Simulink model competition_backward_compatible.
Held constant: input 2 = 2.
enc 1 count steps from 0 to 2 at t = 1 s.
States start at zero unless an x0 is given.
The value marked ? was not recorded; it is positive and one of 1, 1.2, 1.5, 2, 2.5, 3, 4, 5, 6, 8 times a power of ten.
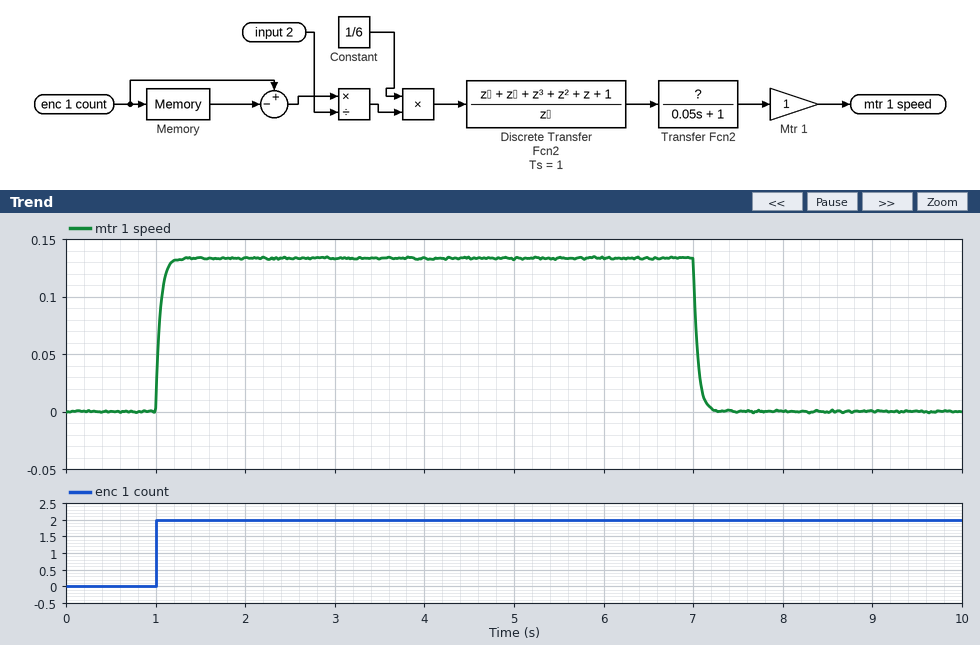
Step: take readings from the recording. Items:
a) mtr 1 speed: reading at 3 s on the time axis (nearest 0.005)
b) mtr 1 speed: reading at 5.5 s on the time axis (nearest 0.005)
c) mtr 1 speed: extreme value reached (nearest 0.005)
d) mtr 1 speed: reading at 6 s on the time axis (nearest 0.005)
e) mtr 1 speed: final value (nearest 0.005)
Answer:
0.135
0.135
0.135
0.135
0.000
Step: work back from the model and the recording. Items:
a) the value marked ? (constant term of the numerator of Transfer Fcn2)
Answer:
0.8
